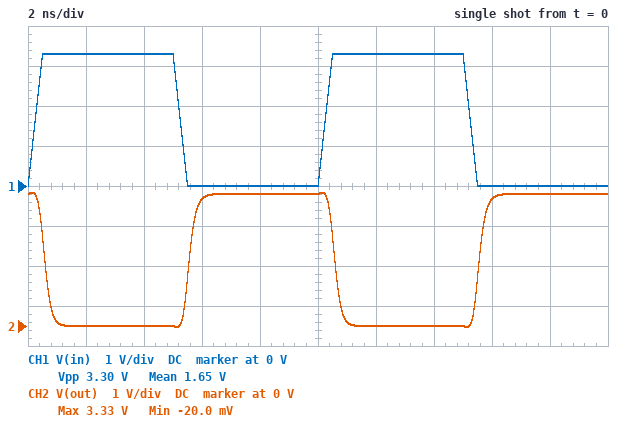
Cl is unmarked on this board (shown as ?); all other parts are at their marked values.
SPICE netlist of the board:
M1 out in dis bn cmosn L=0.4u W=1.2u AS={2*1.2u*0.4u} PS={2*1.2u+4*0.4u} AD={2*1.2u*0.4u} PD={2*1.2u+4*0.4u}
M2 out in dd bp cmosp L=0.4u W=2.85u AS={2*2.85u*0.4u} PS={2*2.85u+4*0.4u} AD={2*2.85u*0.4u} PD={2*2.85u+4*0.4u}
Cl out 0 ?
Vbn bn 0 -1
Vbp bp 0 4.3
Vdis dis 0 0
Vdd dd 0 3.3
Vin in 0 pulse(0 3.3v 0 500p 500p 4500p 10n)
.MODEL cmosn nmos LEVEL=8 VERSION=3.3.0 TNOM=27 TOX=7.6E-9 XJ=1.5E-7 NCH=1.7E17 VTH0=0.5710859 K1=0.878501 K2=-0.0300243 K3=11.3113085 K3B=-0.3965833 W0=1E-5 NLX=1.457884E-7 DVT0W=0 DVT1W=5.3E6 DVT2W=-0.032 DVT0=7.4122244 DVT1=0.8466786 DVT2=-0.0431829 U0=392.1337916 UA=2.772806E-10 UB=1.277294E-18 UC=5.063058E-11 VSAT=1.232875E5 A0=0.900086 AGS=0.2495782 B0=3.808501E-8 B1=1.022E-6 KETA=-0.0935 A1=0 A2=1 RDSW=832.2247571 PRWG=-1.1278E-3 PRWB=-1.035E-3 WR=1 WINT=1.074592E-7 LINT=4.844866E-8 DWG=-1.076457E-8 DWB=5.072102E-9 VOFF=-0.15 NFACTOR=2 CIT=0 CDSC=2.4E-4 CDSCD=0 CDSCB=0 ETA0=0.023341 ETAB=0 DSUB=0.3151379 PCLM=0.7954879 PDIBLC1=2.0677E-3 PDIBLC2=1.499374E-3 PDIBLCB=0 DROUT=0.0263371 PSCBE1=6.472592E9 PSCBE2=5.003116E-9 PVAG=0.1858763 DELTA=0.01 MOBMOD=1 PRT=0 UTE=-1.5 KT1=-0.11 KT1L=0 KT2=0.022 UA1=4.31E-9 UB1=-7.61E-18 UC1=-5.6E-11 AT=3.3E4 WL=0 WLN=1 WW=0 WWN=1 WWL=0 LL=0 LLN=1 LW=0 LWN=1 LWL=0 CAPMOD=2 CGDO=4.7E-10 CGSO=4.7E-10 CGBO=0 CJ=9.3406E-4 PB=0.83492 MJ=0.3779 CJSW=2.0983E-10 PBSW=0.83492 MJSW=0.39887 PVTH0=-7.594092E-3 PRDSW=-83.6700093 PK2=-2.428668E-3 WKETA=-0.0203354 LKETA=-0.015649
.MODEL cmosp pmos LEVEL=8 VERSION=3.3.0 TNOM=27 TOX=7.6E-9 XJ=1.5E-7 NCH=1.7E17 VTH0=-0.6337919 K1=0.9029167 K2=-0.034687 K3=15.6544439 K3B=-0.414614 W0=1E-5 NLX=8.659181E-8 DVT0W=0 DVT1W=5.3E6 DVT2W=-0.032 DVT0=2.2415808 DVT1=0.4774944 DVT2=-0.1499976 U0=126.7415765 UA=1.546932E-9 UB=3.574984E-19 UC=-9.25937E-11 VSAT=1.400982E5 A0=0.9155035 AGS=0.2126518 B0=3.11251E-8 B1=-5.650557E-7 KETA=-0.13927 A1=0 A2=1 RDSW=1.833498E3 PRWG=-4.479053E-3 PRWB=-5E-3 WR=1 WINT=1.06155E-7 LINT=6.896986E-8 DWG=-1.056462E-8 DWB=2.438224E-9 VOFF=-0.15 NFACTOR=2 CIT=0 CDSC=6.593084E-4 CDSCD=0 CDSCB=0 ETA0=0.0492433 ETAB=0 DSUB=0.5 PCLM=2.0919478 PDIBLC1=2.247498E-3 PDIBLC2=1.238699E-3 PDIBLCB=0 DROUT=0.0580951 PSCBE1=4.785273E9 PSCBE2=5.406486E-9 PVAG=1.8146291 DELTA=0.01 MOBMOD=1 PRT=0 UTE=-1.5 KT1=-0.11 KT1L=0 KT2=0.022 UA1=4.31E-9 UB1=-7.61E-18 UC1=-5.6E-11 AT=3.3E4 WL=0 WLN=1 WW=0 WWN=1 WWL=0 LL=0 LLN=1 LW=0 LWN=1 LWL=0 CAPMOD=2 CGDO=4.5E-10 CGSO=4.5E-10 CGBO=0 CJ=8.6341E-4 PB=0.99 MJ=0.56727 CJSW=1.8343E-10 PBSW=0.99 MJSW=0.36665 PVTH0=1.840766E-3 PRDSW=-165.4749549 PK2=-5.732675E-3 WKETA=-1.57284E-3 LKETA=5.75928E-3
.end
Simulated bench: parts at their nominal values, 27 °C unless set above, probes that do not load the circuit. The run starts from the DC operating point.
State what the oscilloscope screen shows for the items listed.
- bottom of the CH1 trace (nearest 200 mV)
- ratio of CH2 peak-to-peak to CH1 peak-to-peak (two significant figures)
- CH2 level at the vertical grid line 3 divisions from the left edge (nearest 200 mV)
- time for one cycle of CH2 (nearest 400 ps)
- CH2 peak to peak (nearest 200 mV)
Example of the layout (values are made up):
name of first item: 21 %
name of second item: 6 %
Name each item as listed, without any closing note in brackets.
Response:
bottom of the CH1 trace: 0 V
ratio of CH2 peak-to-peak to CH1 peak-to-peak: 1.0
CH2 level at the vertical grid line 3 divisions from the left edge: 3.2 V
time for one cycle of CH2: 10.0 ns
CH2 peak to peak: 3.4 V
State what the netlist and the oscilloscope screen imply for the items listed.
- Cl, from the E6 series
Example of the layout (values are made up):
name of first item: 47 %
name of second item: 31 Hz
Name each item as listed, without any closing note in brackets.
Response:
Cl, from the E6 series: 68 fF
